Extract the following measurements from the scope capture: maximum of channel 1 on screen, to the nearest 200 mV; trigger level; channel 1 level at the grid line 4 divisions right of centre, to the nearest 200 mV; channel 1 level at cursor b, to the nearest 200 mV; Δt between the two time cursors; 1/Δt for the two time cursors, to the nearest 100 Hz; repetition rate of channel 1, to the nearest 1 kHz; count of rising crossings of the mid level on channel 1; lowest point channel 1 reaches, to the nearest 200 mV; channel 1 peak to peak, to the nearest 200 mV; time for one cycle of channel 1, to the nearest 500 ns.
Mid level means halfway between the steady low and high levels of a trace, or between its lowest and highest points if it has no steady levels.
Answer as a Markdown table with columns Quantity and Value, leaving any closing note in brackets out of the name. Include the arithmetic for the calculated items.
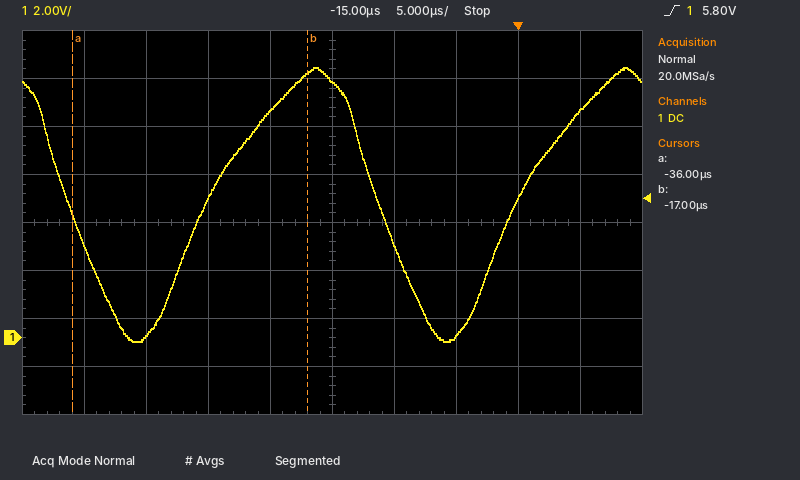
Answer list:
| Quantity | Value |
|---|---|
| maximum of channel 1 on screen, to the nearest 200 mV | 11.2 V |
| trigger level | 5.80 V |
| channel 1 level at the grid line 4 divisions right of centre, to the nearest 200 mV | 9.4 V |
| channel 1 level at cursor b, to the nearest 200 mV | 11.0 V |
| Δt between the two time cursors | -17 µs − (-36 µs) = 19.0 µs |
| 1/Δt for the two time cursors, to the nearest 100 Hz | 1 / 19.0 µs ≈ 52.6 kHz |
| repetition rate of channel 1, to the nearest 1 kHz | 1 / 25.0 µs ≈ 40 kHz |
| count of rising crossings of the mid level on channel 1 | 2 |
| lowest point channel 1 reaches, to the nearest 200 mV | -200 mV |
| channel 1 peak to peak, to the nearest 200 mV | 11.2 V − (-200 mV) = 11.4 V |
| time for one cycle of channel 1, to the nearest 500 ns | 25.0 µs |
